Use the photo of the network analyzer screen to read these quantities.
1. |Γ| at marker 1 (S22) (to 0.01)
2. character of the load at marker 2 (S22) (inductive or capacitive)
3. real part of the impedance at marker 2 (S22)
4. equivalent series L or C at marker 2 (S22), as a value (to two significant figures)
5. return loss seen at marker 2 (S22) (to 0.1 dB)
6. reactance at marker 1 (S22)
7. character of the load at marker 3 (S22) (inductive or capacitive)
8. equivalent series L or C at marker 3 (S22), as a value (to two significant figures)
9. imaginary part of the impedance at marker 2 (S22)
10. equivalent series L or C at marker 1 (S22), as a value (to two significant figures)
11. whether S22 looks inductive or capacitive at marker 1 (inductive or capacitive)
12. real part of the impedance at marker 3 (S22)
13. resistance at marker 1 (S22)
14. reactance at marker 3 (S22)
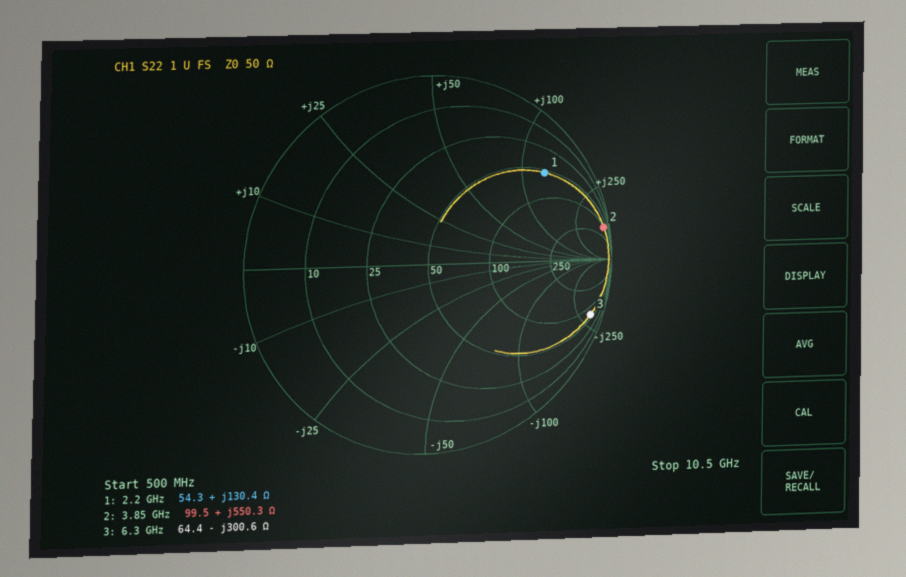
0.78
inductive
99.5 Ω
23 nH
0.3 dB
+130.4 Ω
capacitive
84 fF
+550.3 Ω
9.4 nH
inductive
64.4 Ω
54.3 Ω
-300.6 Ω
